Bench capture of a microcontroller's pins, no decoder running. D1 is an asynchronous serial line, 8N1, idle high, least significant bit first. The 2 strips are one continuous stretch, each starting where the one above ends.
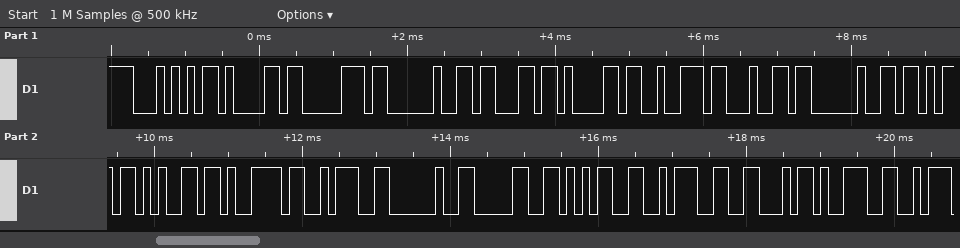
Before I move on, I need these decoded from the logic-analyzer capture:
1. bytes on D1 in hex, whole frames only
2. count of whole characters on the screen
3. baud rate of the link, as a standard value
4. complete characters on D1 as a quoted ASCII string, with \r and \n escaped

0x54 0x61 0x70 0x20 0x63 0x61 0x72 0x64 0x20 0x6B 0x65 0x79 0x3A 0x20 0x30 0x35 0x3A 0x46 0x39
19
9600 baud
"Tap card key: 05:F9"
